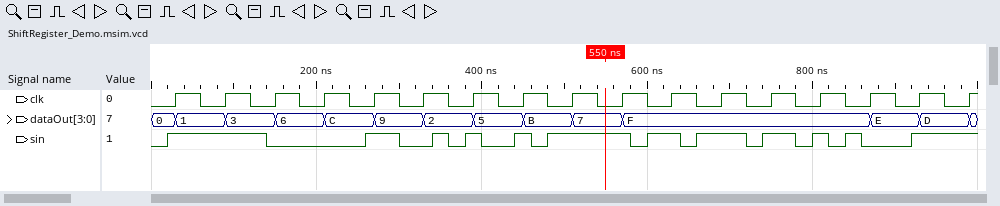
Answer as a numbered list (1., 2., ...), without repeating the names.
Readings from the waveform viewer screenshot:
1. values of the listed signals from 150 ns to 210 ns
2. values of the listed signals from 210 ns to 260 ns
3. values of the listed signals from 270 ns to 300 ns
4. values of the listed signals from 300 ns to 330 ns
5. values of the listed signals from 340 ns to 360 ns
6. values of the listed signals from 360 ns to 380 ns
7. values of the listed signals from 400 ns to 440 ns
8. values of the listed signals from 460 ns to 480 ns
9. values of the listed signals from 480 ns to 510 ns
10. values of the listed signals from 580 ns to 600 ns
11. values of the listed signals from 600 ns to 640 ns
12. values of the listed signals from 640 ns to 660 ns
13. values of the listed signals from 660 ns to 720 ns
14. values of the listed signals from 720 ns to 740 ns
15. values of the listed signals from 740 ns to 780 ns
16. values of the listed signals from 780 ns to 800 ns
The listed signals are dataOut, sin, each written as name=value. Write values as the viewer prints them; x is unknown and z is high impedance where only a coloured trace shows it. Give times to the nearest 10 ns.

1. dataOut=6, sin=0
2. dataOut=C, sin=0
3. dataOut=9, sin=1
4. dataOut=9, sin=0
5. dataOut=2, sin=1
6. dataOut=2, sin=0
7. dataOut=5, sin=0
8. dataOut=B, sin=0
9. dataOut=B, sin=1
10. dataOut=F, sin=0
11. dataOut=F, sin=1
12. dataOut=F, sin=0
13. dataOut=F, sin=1
14. dataOut=F, sin=0
15. dataOut=F, sin=1
16. dataOut=F, sin=0
